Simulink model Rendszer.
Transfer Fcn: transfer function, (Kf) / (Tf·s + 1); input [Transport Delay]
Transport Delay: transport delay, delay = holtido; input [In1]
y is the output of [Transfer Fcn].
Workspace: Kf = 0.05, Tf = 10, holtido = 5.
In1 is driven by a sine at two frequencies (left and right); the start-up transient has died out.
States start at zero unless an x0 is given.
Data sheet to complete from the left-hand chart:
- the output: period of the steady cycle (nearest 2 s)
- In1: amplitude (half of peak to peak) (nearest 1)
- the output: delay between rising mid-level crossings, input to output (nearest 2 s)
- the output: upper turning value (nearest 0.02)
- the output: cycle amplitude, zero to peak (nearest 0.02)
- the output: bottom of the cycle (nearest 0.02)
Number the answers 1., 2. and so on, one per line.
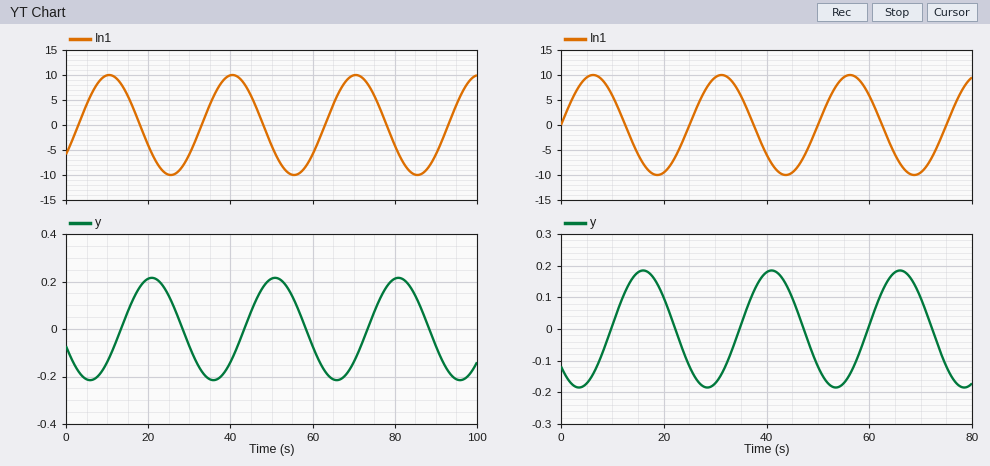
1. 30 s
2. 10
3. 10 s
4. 0.22
5. 0.22
6. -0.22
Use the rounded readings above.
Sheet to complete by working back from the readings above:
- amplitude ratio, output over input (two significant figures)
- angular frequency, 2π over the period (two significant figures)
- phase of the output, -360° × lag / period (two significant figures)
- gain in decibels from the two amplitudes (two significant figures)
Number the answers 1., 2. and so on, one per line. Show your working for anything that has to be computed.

1. 0.22 / 10 = 0.022
2. 2π / 30 = 0.21 rad/s
3. -360 × 10 / 30 = -120°
4. 20 log10(0.22 / 10) = -33 dB
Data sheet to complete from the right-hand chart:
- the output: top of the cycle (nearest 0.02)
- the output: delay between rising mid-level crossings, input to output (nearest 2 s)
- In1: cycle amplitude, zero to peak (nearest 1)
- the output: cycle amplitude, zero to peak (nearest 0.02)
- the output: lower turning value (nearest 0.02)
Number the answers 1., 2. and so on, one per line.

1. 0.18
2. 10 s
3. 10
4. 0.18
5. -0.18
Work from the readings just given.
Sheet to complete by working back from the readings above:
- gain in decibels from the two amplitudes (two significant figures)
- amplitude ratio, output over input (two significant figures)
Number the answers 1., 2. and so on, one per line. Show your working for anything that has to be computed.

1. 20 log10(0.18 / 10) = -35 dB
2. 0.18 / 10 = 0.018
